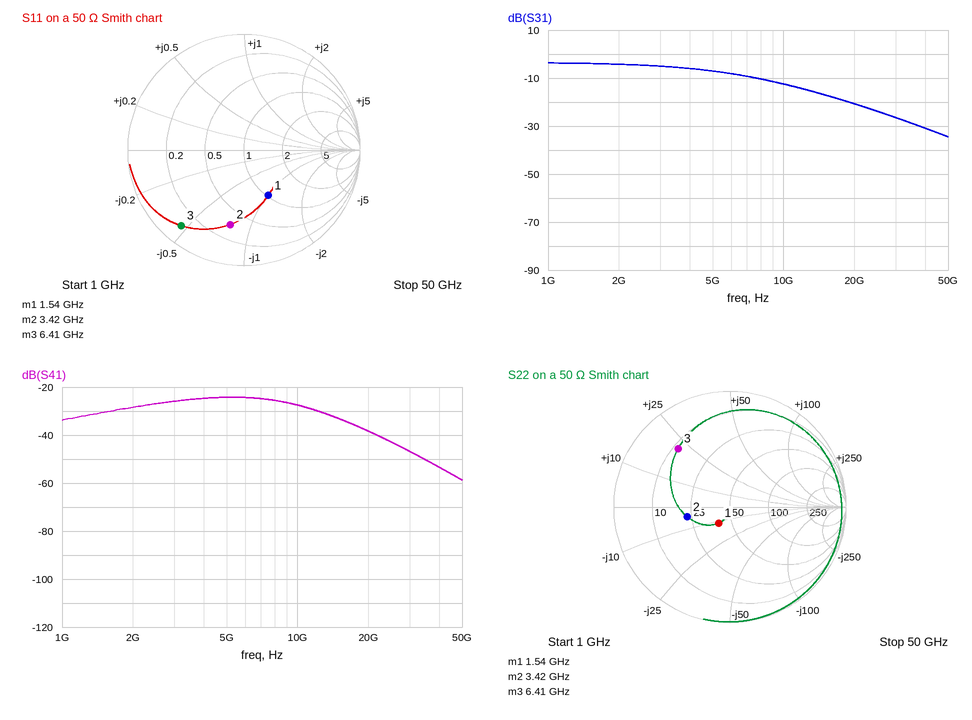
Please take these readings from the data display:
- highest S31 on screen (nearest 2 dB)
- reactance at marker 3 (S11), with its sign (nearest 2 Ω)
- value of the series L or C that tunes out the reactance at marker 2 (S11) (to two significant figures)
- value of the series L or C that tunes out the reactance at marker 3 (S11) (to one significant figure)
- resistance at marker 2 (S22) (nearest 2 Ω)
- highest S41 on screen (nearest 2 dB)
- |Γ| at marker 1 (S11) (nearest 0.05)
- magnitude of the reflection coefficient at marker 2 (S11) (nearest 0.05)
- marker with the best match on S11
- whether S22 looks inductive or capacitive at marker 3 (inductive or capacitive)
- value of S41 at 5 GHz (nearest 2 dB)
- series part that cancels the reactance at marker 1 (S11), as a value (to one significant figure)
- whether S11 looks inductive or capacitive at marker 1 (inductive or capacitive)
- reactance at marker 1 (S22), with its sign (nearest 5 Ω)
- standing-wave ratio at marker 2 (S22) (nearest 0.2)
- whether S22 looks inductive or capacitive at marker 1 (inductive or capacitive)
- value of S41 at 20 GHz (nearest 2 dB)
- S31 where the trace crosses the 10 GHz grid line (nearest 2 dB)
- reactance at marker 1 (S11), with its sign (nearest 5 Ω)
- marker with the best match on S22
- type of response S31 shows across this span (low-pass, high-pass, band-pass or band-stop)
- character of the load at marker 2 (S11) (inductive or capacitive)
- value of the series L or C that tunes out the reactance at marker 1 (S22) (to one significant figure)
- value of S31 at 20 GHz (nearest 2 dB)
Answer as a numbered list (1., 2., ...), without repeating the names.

1. -4 dB
2. -24 Ω
3. 1.8 nH
4. 600 pH
5. 22 Ω
6. -24 dB
7. 0.45
8. 0.65
9. marker 1
10. inductive
11. -24 dB
12. 5 nH
13. capacitive
14. -10 Ω
15. 2.2
16. capacitive
17. -38 dB
18. -12 dB
19. -50 Ω
20. marker 1
21. low-pass
22. capacitive
23. 1 nH
24. -20 dB
